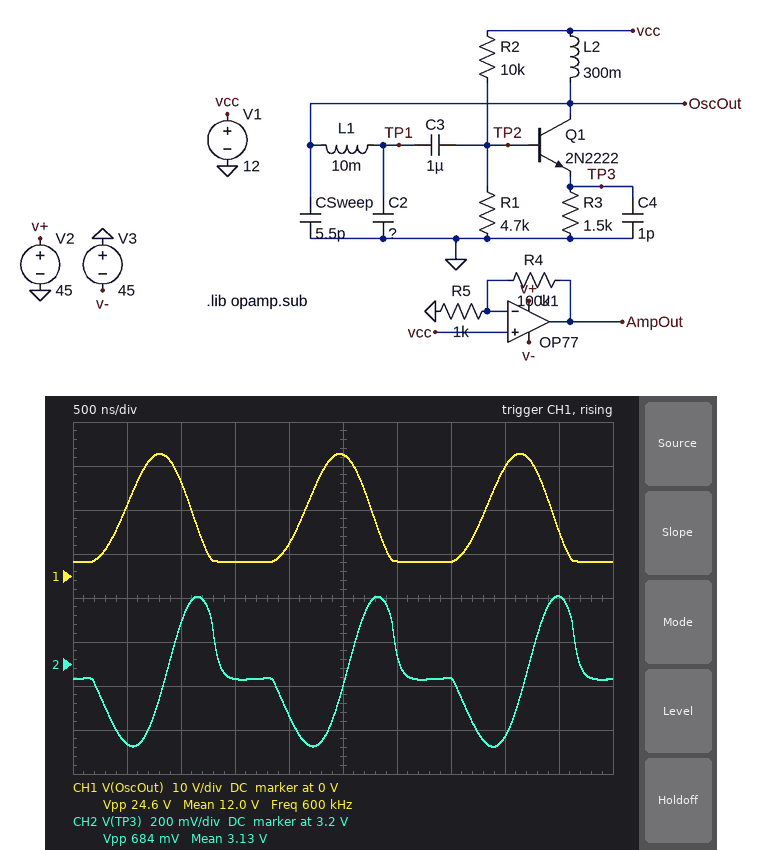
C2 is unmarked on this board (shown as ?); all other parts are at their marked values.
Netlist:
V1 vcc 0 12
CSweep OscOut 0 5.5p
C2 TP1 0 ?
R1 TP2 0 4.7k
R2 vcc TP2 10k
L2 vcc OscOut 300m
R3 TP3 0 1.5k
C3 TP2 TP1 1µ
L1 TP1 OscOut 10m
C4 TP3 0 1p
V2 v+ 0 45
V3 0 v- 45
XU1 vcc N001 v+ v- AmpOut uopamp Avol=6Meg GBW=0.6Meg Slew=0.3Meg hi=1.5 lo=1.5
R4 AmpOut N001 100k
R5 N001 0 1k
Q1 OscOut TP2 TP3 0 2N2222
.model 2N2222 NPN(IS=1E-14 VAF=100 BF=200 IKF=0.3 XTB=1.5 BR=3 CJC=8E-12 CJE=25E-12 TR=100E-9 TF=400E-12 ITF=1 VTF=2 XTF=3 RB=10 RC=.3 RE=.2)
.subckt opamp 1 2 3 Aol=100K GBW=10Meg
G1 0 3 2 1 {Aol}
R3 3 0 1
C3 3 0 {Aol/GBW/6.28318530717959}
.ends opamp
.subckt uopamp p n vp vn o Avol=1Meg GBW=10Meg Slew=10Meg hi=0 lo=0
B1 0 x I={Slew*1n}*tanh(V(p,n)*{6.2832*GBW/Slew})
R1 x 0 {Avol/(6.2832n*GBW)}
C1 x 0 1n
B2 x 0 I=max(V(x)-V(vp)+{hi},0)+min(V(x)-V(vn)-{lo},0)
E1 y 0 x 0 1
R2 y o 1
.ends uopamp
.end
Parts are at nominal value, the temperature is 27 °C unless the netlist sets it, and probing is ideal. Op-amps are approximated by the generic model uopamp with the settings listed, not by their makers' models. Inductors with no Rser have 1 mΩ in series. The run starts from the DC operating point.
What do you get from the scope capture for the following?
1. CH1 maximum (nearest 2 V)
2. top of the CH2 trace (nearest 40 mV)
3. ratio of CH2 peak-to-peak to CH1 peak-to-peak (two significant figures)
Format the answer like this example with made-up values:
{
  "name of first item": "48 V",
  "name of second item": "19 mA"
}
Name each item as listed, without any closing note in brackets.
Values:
{
  "CH1 maximum": "28 V",
  "top of the CH2 trace": "3.52 V",
  "ratio of CH2 peak-to-peak to CH1 peak-to-peak": "0.028"
}
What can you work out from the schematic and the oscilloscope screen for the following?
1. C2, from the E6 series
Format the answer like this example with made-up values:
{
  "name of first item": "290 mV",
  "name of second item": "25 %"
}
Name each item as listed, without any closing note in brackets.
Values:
{
  "C2, from the E6 series": "47 pF"
}
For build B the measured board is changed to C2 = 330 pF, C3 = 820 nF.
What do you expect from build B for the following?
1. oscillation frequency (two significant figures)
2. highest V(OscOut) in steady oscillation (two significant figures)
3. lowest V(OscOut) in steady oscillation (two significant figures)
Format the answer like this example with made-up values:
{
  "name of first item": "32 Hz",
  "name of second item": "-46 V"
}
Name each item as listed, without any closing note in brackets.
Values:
{
  "oscillation frequency": "500 kHz",
  "highest V(OscOut) in steady oscillation": "29 V",
  "lowest V(OscOut) in steady oscillation": "3.2 V"
}
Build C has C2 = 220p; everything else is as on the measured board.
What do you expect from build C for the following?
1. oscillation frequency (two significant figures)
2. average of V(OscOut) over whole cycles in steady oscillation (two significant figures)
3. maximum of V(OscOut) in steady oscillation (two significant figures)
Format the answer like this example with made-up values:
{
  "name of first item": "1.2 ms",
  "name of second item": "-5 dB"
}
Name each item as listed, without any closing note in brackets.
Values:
{
  "oscillation frequency": "510 kHz",
  "average of V(OscOut) over whole cycles in steady oscillation": "12 V",
  "maximum of V(OscOut) in steady oscillation": "29 V"
}
